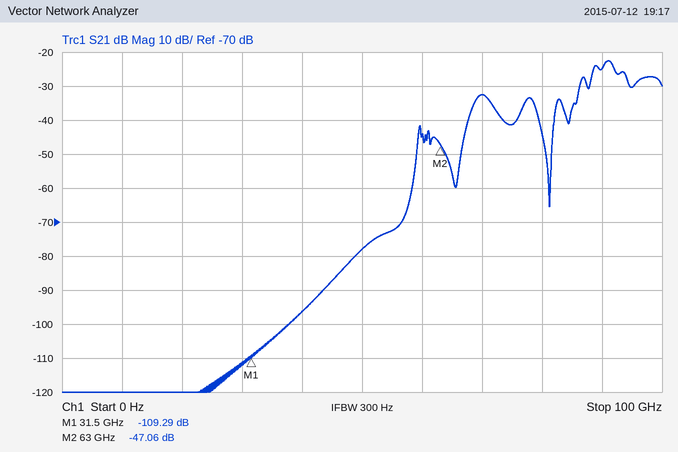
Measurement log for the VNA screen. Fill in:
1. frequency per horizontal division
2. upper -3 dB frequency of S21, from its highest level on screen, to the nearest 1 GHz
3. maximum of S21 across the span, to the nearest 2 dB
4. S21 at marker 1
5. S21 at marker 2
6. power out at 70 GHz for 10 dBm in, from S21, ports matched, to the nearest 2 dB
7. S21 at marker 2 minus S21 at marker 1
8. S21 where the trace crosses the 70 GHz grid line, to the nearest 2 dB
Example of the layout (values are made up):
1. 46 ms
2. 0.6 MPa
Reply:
1. 10 GHz
2. 92 GHz
3. -22 dB
4. -109.29 dB
5. -47.06 dB
6. -22 dBm
7. 62.23 dB
8. -32 dB
